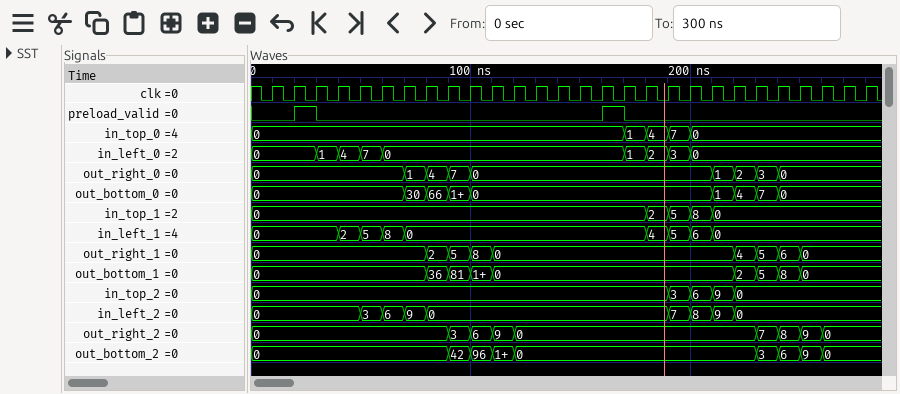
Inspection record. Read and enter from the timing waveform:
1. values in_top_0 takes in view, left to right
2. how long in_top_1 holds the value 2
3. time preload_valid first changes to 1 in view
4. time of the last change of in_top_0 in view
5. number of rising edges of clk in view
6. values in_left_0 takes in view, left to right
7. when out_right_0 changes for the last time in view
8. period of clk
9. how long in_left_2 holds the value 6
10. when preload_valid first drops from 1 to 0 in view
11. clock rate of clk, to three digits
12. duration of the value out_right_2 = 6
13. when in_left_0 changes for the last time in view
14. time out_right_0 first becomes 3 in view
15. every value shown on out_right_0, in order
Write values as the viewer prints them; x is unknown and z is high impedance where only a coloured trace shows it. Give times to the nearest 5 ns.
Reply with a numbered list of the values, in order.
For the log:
1. 0, 1, 4, 7, 0
2. 10 ns
3. 20 ns
4. 200 ns
5. 28
6. 0, 1, 4, 7, 0, 1, 2, 3, 0
7. 240 ns
8. 10 ns
9. 10 ns
10. 30 ns
11. 100 MHz
12. 10 ns
13. 200 ns
14. 230 ns
15. 0, 1, 4, 7, 0, 1, 2, 3, 0
